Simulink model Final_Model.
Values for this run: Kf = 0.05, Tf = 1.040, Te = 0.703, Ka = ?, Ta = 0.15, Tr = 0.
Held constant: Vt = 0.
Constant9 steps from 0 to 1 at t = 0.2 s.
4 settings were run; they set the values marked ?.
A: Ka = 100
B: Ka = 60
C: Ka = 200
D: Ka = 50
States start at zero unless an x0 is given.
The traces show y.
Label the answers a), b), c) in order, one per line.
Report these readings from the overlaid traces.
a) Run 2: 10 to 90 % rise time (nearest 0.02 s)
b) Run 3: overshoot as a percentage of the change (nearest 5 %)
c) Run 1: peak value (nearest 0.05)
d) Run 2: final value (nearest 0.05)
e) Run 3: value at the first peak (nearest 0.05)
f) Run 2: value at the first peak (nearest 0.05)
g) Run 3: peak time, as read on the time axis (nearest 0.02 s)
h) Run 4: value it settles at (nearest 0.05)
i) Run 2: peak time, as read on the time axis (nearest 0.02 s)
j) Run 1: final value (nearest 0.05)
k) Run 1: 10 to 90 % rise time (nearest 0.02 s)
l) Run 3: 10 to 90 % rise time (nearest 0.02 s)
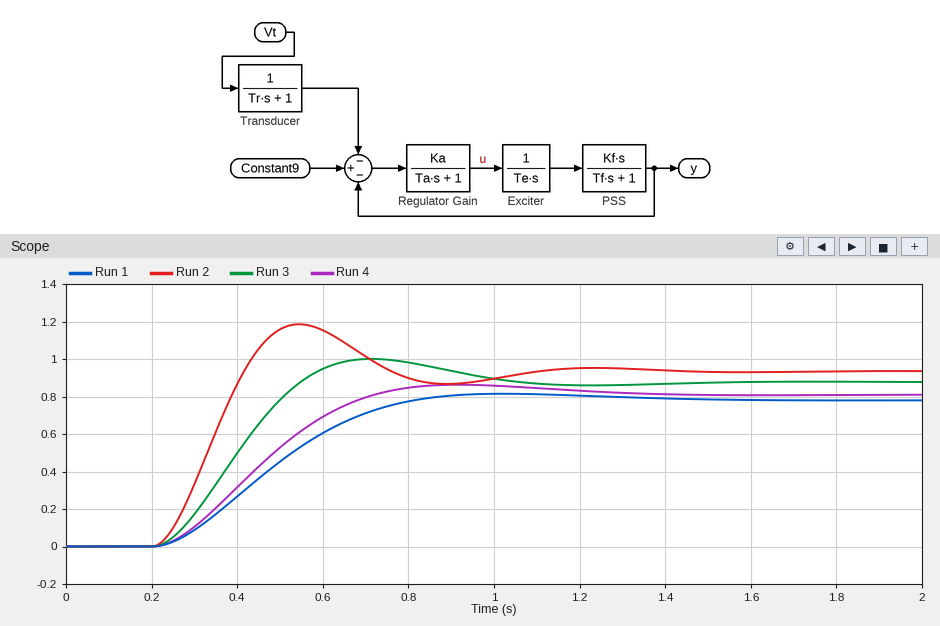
a) 0.14 s
b) 15 %
c) 0.80
d) 0.95
e) 1.00
f) 1.20
g) 0.72 s
h) 0.80
i) 0.54 s
j) 0.80
k) 0.40 s
l) 0.24 s
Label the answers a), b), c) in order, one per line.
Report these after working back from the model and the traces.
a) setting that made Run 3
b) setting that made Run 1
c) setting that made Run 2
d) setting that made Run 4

a) A
b) D
c) C
d) B
